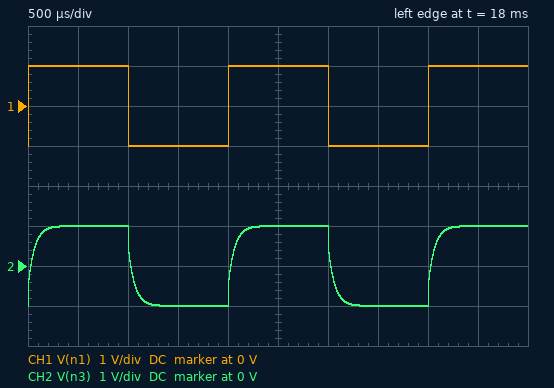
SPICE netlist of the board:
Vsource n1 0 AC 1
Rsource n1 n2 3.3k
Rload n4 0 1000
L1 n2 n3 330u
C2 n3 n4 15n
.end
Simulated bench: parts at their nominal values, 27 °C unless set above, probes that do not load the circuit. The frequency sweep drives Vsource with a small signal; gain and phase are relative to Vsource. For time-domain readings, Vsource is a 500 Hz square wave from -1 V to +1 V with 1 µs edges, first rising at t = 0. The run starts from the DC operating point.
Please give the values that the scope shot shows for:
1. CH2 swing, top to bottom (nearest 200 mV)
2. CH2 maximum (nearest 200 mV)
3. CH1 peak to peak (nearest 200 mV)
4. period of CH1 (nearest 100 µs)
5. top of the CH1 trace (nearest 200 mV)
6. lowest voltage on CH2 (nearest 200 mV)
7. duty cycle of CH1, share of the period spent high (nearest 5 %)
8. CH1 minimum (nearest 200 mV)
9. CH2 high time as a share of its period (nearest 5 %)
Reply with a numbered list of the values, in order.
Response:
1. 2.0 V
2. 1.0 V
3. 2.0 V
4. 2.0 ms
5. 1.0 V
6. -1.0 V
7. 50 %
8. -1.0 V
9. 50 %
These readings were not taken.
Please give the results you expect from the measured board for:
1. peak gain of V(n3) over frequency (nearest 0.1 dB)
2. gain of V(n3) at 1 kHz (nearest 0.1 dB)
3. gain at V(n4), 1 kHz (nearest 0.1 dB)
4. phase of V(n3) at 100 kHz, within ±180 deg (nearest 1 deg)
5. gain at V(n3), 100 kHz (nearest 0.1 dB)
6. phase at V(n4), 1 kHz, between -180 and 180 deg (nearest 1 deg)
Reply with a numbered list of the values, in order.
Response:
1. 0 dB
2. -0.6 dB
3. -21.2 dB
4. -7 deg
5. -12.6 dB
6. 68 deg
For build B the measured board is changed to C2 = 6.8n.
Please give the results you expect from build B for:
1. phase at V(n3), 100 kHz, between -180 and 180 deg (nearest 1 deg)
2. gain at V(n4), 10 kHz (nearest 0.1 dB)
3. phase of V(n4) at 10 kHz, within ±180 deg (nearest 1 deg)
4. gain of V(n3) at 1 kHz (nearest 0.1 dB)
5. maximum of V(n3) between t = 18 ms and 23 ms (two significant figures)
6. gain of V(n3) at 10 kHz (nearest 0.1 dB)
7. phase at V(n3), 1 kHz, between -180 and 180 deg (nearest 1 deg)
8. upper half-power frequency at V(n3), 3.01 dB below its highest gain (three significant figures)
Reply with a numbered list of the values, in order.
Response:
1. -13 deg
2. -13.8 dB
3. 28 deg
4. -0.1 dB
5. 1.0 V
6. -5.7 dB
7. -8 deg
8. 5.78 kHz
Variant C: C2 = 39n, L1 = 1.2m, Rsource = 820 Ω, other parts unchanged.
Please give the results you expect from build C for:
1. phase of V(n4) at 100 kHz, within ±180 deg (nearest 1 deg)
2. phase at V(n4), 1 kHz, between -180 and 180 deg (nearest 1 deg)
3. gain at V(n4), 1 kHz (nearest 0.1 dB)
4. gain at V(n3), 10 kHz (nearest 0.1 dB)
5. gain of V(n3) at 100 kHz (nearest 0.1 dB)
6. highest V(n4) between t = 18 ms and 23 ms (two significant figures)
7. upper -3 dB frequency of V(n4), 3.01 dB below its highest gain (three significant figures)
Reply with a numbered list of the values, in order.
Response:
1. -21 deg
2. 66 deg
3. -13.0 dB
4. -4.7 dB
5. -5.8 dB
6. 1.1 V
7. 244 kHz
